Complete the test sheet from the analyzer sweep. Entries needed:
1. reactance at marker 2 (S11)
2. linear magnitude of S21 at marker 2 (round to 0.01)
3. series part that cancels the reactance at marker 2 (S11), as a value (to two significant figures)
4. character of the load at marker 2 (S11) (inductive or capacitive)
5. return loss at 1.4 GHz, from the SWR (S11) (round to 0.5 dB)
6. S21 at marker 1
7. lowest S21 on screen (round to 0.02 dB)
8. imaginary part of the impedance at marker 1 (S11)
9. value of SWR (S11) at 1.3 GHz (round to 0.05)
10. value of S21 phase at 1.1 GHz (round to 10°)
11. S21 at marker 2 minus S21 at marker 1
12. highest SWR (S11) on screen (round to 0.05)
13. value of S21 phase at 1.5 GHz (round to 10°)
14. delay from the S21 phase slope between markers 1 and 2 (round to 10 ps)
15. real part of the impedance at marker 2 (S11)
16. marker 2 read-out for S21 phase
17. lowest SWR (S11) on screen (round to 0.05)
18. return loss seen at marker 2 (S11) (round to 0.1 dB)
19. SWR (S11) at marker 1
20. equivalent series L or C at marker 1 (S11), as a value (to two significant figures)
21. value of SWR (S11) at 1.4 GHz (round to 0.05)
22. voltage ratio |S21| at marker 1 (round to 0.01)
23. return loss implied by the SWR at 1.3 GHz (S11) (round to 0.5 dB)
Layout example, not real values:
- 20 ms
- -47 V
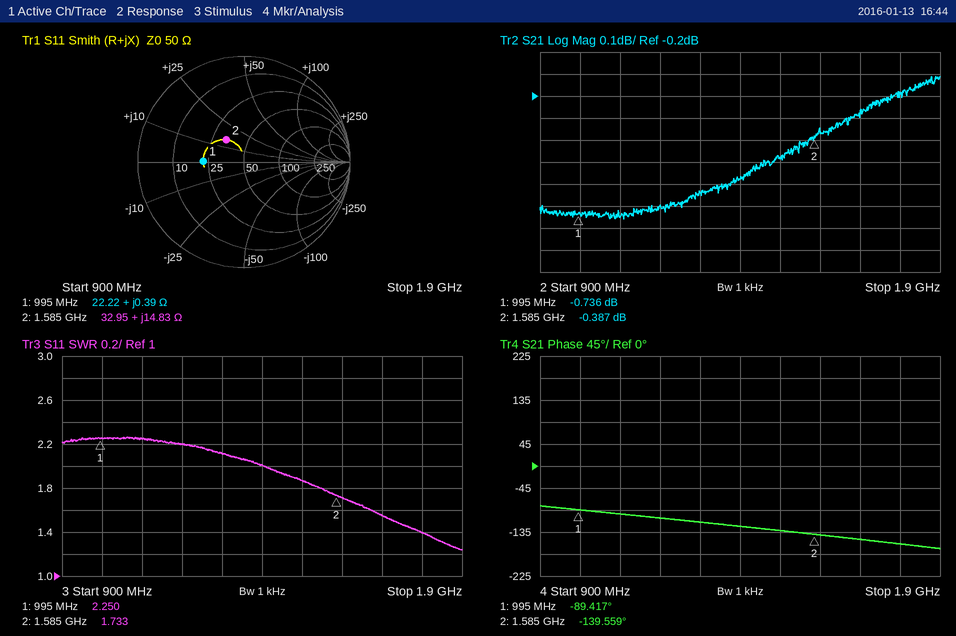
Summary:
- +14.83 Ω
- 0.96
- 6.8 pF
- inductive
- 9.5 dB
- -0.736 dB
- -0.76 dB
- +0.39 Ω
- 2.10
- -100°
- 0.349 dB
- 2.25
- -130°
- 240 ps
- 32.95 Ω
- -139.559°
- 1.25
- 11.4 dB
- 2.250
- 62 pH
- 2.00
- 0.92
- 9.0 dB
